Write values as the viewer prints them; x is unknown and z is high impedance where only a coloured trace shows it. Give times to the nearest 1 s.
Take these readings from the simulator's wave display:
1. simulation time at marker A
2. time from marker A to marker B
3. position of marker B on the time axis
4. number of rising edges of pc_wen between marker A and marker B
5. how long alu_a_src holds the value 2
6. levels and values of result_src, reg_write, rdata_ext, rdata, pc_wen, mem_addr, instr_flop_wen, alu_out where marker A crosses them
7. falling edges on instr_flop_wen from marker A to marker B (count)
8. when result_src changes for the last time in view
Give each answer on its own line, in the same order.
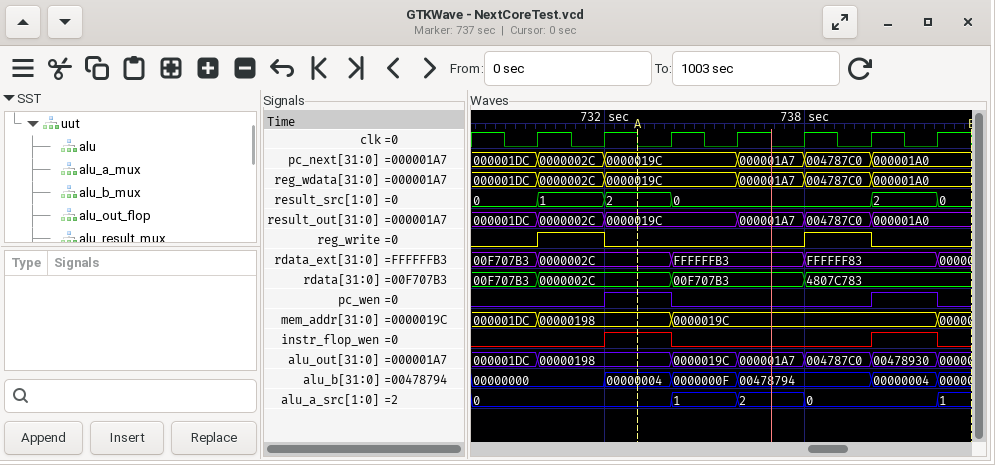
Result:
733 s
10 s
743 s
1
2 s
result_src=2, reg_write=0, rdata_ext=0000002C, rdata=0000002C, pc_wen=1, mem_addr=00000198, instr_flop_wen=1, alu_out=00000198
2
742 s
